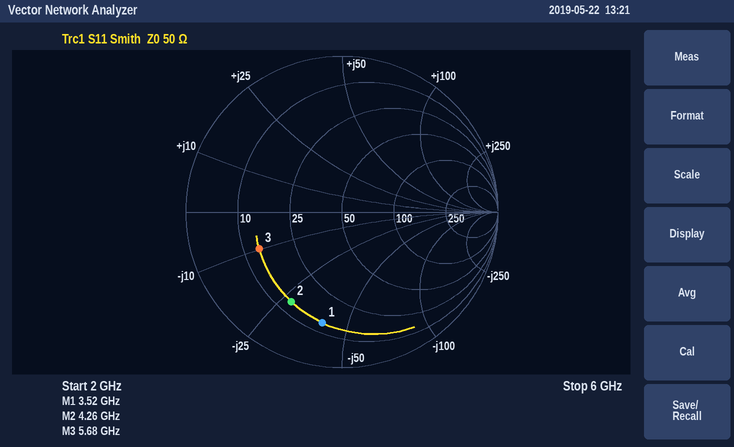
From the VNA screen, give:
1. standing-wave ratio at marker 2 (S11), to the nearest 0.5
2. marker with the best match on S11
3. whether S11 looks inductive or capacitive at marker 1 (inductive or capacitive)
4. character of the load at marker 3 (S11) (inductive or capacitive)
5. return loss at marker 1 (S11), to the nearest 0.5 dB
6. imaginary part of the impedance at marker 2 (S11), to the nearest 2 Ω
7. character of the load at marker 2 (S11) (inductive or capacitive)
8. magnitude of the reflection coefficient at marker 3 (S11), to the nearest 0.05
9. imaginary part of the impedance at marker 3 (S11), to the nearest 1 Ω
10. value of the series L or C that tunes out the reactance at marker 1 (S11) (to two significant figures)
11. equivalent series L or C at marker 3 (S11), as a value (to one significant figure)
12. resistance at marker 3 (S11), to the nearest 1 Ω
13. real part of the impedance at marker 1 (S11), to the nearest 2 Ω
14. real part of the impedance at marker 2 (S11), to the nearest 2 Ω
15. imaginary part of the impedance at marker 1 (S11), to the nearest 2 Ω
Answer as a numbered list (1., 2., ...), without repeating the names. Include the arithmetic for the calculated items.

1. 5.0
2. marker 3
3. capacitive
4. capacitive
5. 3.0 dB
6. -28 Ω
7. capacitive
8. 0.60
9. -10 Ω
10. L = 40 Ω/(2π × 3.52 GHz) ≈ 1.8 nH
11. C = 1/(2π × 5.68 GHz × 10 Ω) ≈ 3 pF
12. 14 Ω
13. 14 Ω
14. 14 Ω
15. -40 Ω
